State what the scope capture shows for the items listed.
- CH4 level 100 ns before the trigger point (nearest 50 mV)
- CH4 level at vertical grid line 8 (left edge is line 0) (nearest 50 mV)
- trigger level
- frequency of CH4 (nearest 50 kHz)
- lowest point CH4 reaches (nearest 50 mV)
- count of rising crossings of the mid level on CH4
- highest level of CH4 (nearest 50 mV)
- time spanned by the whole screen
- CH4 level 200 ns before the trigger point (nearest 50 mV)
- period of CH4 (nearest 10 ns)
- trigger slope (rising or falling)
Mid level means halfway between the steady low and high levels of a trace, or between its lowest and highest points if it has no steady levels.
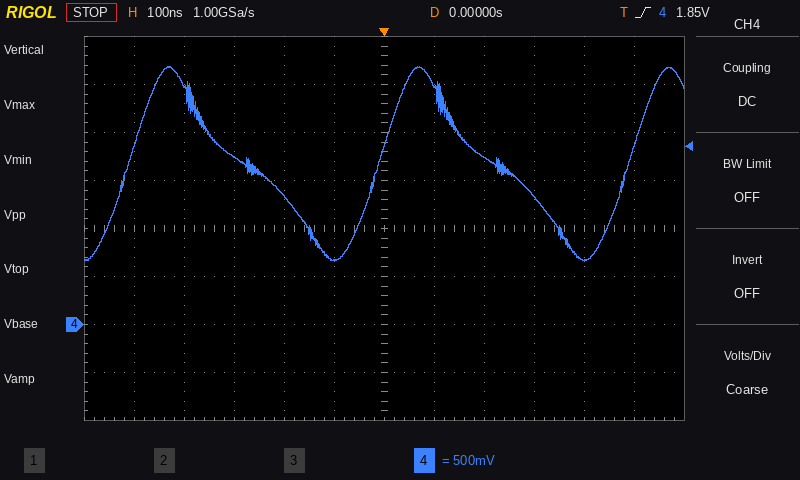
650 mV
1.75 V
1.85 V
2.00 MHz
650 mV
3
2.70 V
1.2 µs
1.35 V
500 ns
rising
